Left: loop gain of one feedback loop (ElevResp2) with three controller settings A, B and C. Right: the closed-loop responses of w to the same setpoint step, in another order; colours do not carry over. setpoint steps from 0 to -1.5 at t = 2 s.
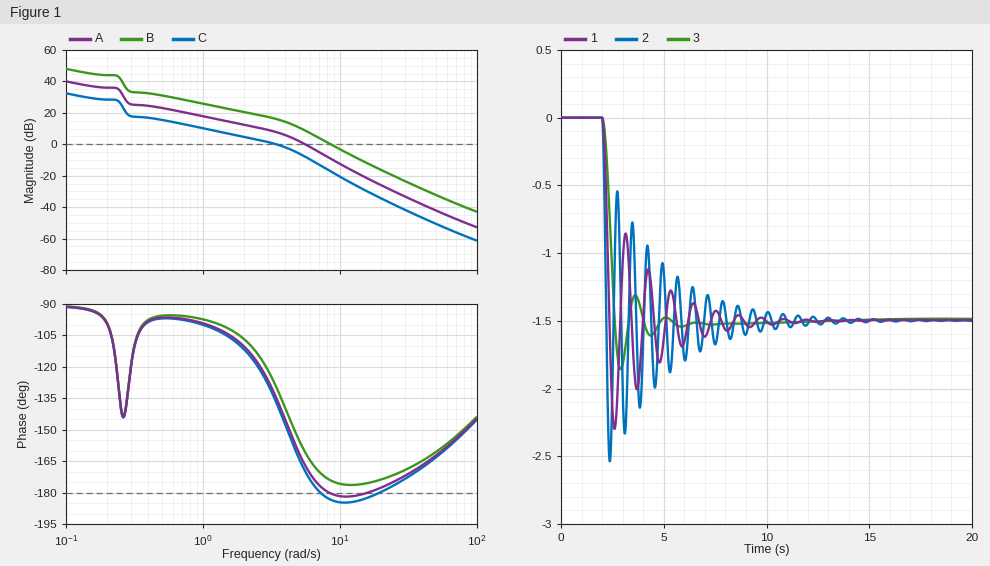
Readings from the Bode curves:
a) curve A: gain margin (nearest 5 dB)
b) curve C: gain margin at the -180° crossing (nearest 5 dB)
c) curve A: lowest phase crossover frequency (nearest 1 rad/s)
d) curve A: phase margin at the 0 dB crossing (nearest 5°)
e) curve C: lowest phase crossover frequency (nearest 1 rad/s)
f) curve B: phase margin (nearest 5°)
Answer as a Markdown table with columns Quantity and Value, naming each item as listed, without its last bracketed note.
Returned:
| Quantity | Value |
|---|---|
| curve A: gain margin | 10 dB |
| curve C: gain margin at the -180° crossing | 15 dB |
| curve A: lowest phase crossover frequency | 8 rad/s |
| curve A: phase margin at the 0 dB crossing | 15° |
| curve C: lowest phase crossover frequency | 7 rad/s |
| curve B: phase margin | 5° |
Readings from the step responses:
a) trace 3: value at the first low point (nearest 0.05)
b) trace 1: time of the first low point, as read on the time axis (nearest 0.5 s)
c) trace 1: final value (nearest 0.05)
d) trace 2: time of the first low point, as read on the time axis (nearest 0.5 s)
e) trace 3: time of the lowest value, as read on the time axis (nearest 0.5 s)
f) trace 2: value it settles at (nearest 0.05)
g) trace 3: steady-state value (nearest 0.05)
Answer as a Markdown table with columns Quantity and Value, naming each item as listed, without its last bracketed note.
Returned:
| Quantity | Value |
|---|---|
| trace 3: value at the first low point | -1.85 |
| trace 1: time of the first low point, as read on the time axis | 2.5 s |
| trace 1: final value | -1.50 |
| trace 2: time of the first low point, as read on the time axis | 2.5 s |
| trace 3: time of the lowest value, as read on the time axis | 3.0 s |
| trace 2: value it settles at | -1.50 |
| trace 3: steady-state value | -1.50 |
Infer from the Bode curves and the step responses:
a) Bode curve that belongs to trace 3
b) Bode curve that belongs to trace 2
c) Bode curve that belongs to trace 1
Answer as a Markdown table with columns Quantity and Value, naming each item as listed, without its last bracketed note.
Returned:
| Quantity | Value |
|---|---|
| Bode curve that belongs to trace 3 | C |
| Bode curve that belongs to trace 2 | B |
| Bode curve that belongs to trace 1 | A |
